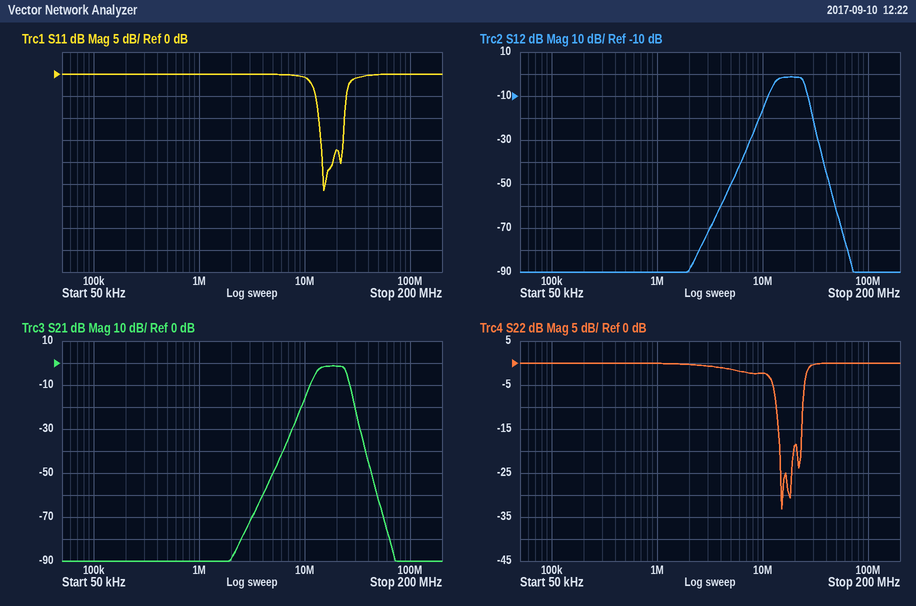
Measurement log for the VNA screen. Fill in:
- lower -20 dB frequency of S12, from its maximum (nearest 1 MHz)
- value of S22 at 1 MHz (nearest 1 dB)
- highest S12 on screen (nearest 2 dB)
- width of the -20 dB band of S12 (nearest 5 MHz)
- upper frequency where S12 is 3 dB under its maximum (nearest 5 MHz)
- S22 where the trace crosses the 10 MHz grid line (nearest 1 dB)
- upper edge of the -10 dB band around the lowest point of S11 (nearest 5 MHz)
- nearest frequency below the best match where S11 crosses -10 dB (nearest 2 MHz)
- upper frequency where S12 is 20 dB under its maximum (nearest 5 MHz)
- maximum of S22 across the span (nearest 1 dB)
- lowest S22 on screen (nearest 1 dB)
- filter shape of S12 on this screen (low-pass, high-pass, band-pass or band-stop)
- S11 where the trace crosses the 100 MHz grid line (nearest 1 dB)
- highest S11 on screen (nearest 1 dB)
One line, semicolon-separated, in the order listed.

9 MHz; 0 dB; -2 dB; 20 MHz; 25 MHz; -2 dB; 25 MHz; 14 MHz; 30 MHz; 0 dB; -33 dB; band-pass; 0 dB; 0 dB
